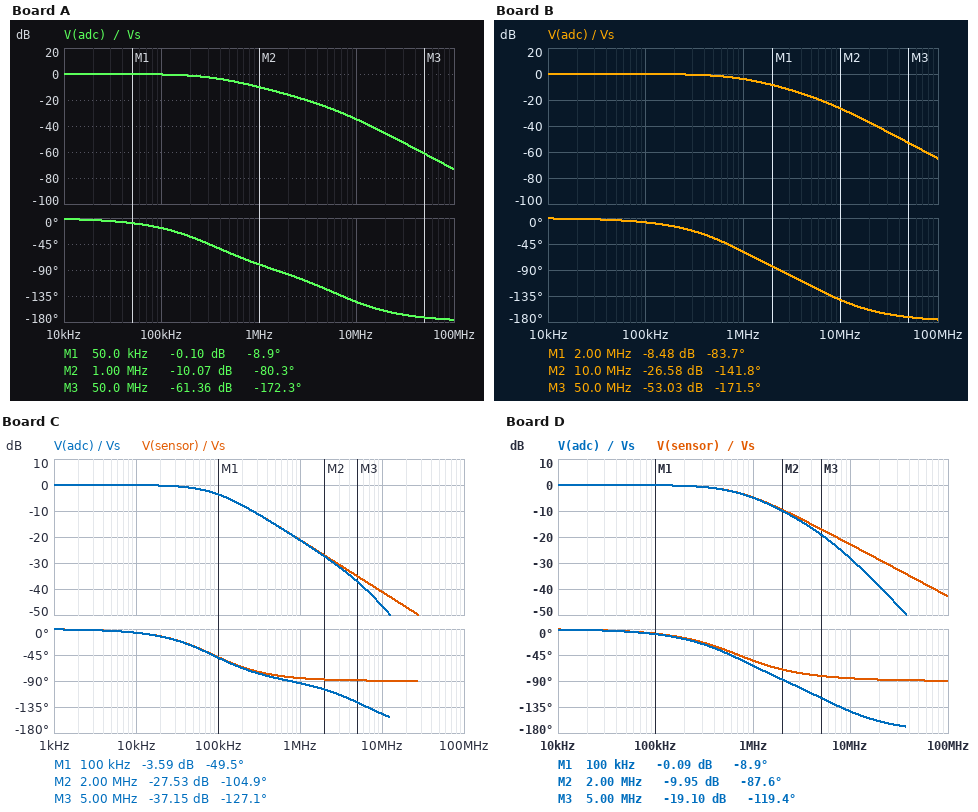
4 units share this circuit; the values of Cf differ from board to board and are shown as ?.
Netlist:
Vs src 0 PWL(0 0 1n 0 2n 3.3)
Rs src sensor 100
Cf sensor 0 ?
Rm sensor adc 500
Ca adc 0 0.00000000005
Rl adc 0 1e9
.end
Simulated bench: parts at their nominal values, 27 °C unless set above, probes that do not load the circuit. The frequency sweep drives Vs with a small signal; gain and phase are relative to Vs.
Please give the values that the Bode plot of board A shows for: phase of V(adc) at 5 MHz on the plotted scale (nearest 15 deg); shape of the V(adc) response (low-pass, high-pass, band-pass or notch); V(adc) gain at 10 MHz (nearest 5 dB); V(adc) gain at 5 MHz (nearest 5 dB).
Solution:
-120 deg
low-pass
-35 dB
-25 dB
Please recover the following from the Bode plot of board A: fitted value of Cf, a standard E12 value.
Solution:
4.7 nF
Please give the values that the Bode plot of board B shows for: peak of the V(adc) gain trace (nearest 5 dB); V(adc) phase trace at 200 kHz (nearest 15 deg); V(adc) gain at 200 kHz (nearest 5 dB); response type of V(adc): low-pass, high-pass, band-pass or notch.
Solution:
0 dB
-15 deg
0 dB
low-pass
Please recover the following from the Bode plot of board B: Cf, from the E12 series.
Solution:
1.8 nF
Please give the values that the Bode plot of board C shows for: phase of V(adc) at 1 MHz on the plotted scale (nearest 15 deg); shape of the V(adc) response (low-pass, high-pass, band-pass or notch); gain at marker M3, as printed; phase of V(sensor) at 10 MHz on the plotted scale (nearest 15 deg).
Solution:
-90 deg
low-pass
-37.15 dB
-90 deg
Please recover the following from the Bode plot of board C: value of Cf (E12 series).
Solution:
18 nF
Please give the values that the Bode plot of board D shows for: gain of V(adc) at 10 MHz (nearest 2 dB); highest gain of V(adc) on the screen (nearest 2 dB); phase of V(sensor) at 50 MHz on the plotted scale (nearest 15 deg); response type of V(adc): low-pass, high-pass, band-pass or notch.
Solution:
-28 dB
0 dB
-90 deg
low-pass
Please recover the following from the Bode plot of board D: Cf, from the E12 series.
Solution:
2.2 nF
